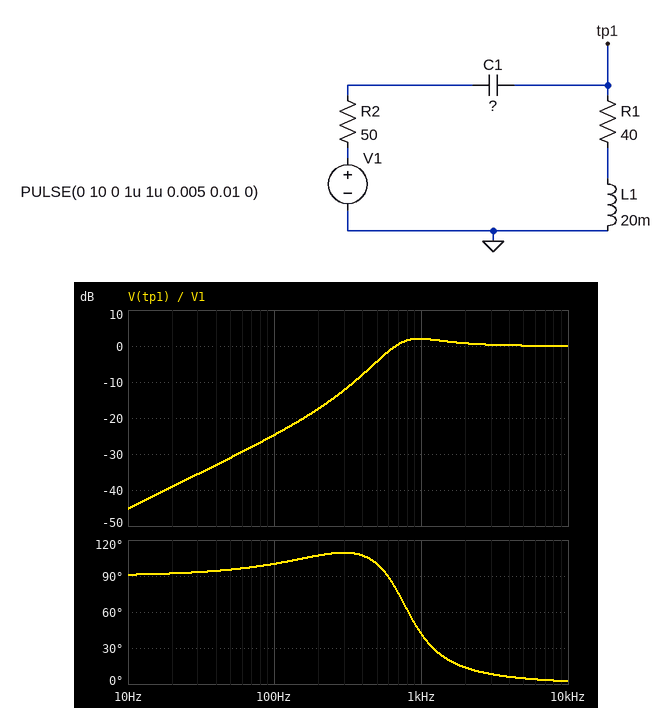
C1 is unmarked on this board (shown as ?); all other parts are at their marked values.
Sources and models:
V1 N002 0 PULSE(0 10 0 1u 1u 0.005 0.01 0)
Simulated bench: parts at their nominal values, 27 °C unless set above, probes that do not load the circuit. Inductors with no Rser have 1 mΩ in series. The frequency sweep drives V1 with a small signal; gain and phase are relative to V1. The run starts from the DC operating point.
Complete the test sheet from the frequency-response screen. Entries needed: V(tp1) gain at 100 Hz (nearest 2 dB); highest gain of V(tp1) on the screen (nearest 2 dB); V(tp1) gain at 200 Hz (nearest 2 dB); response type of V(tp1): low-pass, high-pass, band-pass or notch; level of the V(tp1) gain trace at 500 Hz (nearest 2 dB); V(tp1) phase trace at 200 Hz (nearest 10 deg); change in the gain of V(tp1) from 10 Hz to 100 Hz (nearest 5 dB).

-24 dB
2 dB
-18 dB
high-pass
-4 dB
110 deg
20 dB
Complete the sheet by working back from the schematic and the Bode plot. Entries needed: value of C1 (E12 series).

2.2 µF
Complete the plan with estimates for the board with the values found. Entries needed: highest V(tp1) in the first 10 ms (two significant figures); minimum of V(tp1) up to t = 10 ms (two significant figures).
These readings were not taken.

10 V
-10 V
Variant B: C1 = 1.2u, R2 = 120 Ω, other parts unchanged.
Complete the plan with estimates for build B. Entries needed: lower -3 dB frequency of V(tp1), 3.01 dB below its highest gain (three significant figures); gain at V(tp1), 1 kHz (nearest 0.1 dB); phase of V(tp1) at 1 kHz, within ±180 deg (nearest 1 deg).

903 Hz
-1.7 dB
75 deg
